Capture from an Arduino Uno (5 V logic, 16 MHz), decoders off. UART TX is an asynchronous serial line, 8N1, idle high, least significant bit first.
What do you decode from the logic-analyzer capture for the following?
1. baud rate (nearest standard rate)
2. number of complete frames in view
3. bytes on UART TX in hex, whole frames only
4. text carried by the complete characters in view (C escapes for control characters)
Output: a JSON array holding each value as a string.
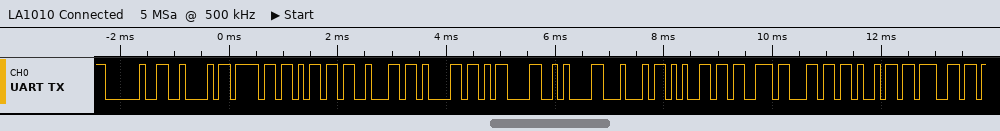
["9600 baud", "14", "0x20 0x42 0x6F 0x6D 0x62 0x61 0x0D 0x0A 0x44 0x65 0x73 0x6C 0x69 0x67", "\" Bomba\\r\\nDeslig\""]
